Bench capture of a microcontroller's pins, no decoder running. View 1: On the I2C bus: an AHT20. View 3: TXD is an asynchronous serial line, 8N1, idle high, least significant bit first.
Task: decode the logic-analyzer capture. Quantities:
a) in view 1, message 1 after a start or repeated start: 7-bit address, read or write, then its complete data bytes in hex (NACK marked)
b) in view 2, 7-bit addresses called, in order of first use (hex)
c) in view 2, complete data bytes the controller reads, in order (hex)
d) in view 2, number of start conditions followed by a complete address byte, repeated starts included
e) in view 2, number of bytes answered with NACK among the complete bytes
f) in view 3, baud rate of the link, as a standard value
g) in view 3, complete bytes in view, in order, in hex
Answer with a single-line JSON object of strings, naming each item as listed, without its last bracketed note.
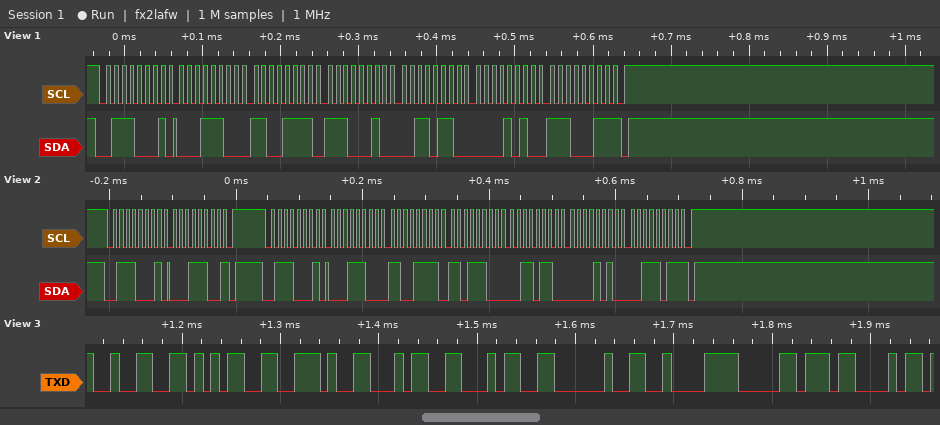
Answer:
{"in view 1, message 1 after a start or repeated start: 7-bit address, read or write, then its complete data bytes in hex": "0x38 read: 1C CF E2 36 0A E3 NACK", "in view 2, 7-bit addresses called, in order of first use": "0x38", "in view 2, complete data bytes the controller reads, in order": "1C 1C CF DC 36 0A 3B", "in view 2, number of start conditions followed by a complete address byte, repeated starts included": "2", "in view 2, number of bytes answered with NACK among the complete bytes": "2", "in view 3, baud rate of the link, as a standard value": "115200 baud", "in view 3, complete bytes in view, in order, in hex": "0x32 0x35 0x2E 0x34 0x34 0x20 0xC2 0xB0 0x43"}
